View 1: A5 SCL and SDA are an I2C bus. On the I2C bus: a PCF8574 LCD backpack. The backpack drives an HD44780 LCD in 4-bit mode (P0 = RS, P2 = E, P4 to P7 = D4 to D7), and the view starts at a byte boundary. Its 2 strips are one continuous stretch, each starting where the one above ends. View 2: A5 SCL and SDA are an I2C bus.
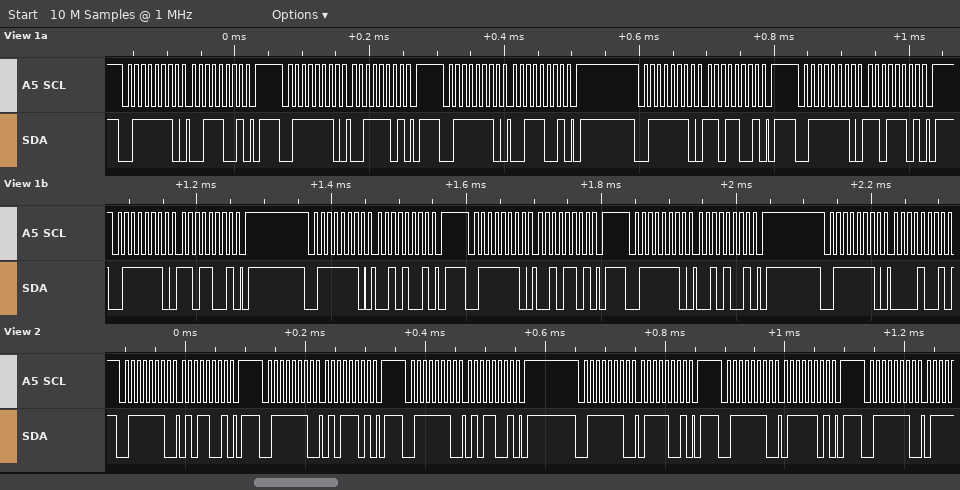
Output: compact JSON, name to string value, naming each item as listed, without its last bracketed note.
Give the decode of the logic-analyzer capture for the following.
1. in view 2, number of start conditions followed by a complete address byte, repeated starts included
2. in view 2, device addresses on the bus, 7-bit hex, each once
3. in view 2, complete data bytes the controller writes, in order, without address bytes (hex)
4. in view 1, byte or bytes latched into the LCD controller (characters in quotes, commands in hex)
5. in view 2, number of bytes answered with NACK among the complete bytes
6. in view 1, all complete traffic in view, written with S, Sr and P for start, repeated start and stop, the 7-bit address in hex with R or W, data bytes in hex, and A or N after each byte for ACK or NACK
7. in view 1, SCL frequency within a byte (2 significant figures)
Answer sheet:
{"in view 2, number of start conditions followed by a complete address byte, repeated starts included": "6", "in view 2, device addresses on the bus, 7-bit hex, each once": "0x3F", "in view 2, complete data bytes the controller writes, in order, without address bytes": "59 5D 59 79 7D", "in view 1, byte or bytes latched into the LCD controller": "'='", "in view 2, number of bytes answered with NACK among the complete bytes": "0", "in view 1, all complete traffic in view, written with S, Sr and P for start, repeated start and stop, the 7-bit address in hex with R or W, data bytes in hex, and A or N after each byte for ACK or NACK": "S 3FW A 39 A P S 3FW A 3D A P S 3FW A 39 A P S 3FW A D9 A P S 3FW A DD A P S 3FW A D9 A P S 3FW A 29 A P S 3FW A 2D A P S 3FW A 29 A P S 3FW A 09 A", "in view 1, SCL frequency within a byte": "100 kHz"}
